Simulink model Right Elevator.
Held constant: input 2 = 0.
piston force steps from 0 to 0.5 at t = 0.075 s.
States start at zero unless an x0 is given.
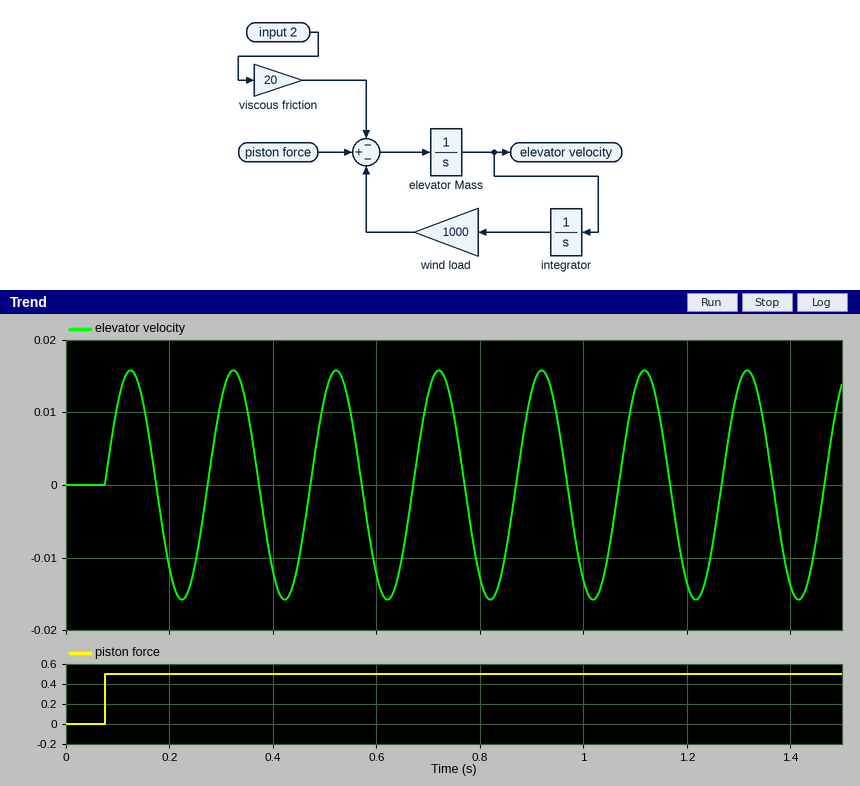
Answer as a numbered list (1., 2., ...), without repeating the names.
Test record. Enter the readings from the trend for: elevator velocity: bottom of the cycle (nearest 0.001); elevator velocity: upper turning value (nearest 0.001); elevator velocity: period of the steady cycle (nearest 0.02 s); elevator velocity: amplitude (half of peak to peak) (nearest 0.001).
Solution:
1. -0.016
2. 0.016
3. 0.20 s
4. 0.016
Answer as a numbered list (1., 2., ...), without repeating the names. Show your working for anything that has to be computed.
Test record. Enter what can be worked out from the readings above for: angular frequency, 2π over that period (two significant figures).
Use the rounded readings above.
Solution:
1. 2π / 0.2 = 31 rad/s
